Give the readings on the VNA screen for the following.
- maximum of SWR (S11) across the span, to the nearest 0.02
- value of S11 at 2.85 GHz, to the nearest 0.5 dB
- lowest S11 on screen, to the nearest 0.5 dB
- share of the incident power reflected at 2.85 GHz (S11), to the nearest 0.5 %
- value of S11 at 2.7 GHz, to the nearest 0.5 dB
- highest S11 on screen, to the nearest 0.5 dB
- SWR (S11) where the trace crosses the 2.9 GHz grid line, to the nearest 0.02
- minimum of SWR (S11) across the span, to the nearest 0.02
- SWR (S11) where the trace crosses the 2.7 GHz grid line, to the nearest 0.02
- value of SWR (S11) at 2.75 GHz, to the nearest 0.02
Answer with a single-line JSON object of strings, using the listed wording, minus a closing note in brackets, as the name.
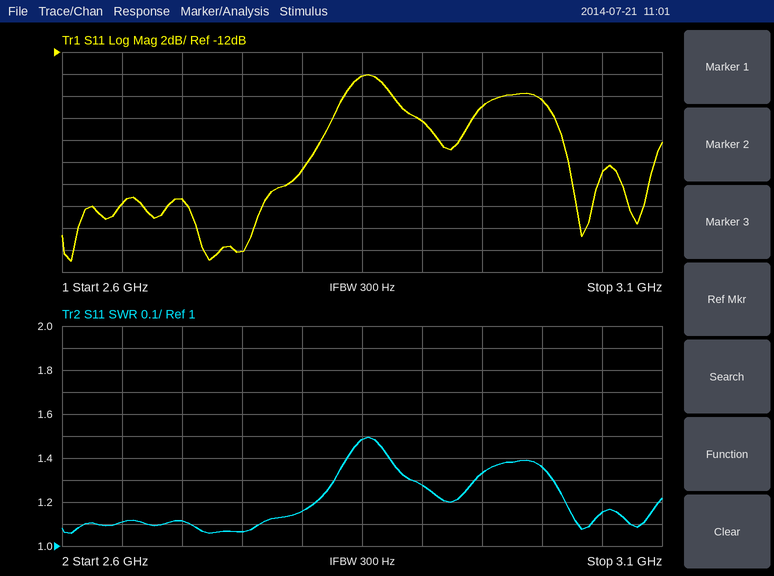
{"maximum of SWR (S11) across the span, to the nearest 0.02": "1.50", "value of S11 at 2.85 GHz, to the nearest 0.5 dB": "-14.0 dB", "lowest S11 on screen, to the nearest 0.5 dB": "-31.0 dB", "share of the incident power reflected at 2.85 GHz (S11), to the nearest 0.5 %": "4.0 %", "value of S11 at 2.7 GHz, to the nearest 0.5 dB": "-25.5 dB", "highest S11 on screen, to the nearest 0.5 dB": "-14.0 dB", "SWR (S11) where the trace crosses the 2.9 GHz grid line, to the nearest 0.02": "1.28", "minimum of SWR (S11) across the span, to the nearest 0.02": "1.06", "SWR (S11) where the trace crosses the 2.7 GHz grid line, to the nearest 0.02": "1.12", "value of SWR (S11) at 2.75 GHz, to the nearest 0.02": "1.06"}
